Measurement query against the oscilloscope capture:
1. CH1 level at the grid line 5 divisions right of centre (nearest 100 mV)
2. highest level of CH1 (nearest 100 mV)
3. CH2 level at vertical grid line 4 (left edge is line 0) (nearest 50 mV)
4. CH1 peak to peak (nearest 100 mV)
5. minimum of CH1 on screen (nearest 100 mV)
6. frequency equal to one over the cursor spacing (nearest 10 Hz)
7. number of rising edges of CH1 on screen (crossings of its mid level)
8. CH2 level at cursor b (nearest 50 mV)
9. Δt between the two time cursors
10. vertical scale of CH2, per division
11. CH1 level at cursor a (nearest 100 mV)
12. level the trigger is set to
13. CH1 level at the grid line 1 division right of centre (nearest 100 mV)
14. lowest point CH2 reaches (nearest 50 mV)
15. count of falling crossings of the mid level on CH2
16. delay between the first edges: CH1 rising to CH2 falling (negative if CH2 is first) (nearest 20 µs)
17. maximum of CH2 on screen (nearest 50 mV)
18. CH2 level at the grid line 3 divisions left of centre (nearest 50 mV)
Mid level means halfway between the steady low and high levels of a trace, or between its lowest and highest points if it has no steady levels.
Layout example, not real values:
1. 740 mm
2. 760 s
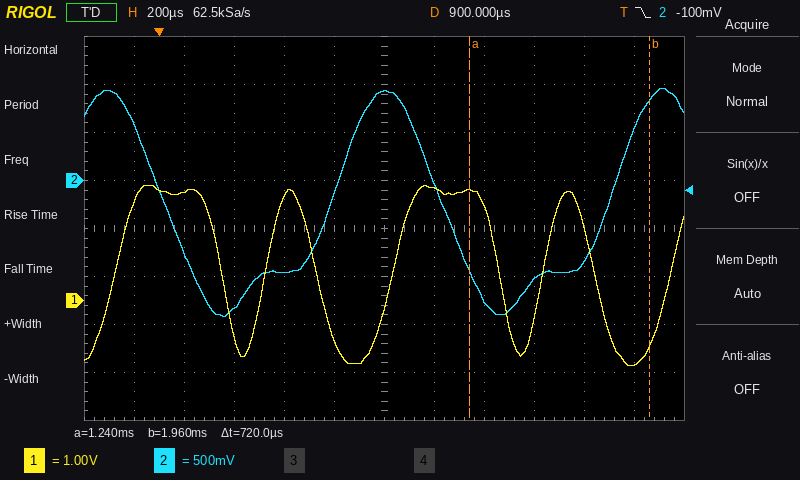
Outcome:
1. -1.3 V
2. 2.4 V
3. -950 mV
4. 3.8 V
5. -1.4 V
6. 1.39 kHz
7. 5
8. 850 mV
9. 720 µs
10. 500 mV
11. 2.3 V
12. -100 mV
13. 2.3 V
14. -1.40 V
15. 2
16. +200 µs
17. 950 mV
18. -1.35 V
